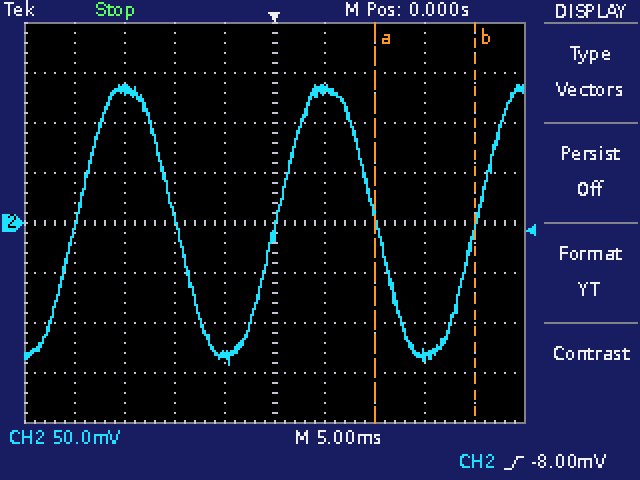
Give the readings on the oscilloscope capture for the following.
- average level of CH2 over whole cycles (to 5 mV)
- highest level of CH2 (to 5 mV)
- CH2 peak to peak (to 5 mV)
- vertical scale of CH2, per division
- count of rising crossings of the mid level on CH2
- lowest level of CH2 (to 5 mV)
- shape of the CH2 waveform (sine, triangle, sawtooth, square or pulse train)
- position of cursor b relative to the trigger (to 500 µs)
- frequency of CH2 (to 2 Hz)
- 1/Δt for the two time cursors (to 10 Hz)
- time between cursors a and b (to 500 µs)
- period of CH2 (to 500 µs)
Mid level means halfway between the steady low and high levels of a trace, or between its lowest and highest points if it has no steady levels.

0 mV
140 mV
280 mV
50 mV
3
-140 mV
sine
+20.0 ms
50 Hz
100 Hz
10.0 ms
20.0 ms
